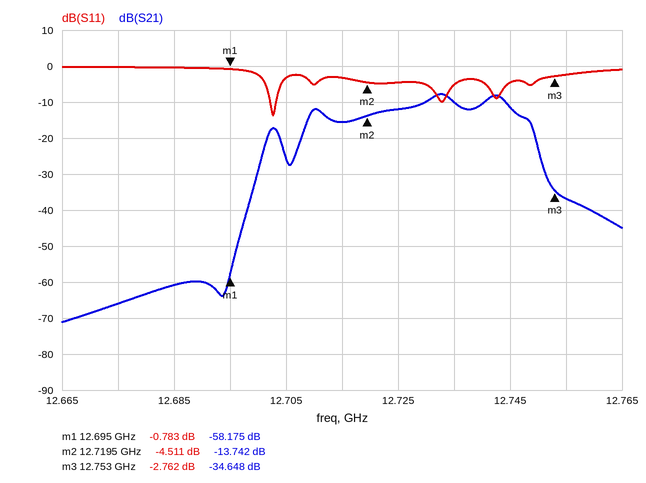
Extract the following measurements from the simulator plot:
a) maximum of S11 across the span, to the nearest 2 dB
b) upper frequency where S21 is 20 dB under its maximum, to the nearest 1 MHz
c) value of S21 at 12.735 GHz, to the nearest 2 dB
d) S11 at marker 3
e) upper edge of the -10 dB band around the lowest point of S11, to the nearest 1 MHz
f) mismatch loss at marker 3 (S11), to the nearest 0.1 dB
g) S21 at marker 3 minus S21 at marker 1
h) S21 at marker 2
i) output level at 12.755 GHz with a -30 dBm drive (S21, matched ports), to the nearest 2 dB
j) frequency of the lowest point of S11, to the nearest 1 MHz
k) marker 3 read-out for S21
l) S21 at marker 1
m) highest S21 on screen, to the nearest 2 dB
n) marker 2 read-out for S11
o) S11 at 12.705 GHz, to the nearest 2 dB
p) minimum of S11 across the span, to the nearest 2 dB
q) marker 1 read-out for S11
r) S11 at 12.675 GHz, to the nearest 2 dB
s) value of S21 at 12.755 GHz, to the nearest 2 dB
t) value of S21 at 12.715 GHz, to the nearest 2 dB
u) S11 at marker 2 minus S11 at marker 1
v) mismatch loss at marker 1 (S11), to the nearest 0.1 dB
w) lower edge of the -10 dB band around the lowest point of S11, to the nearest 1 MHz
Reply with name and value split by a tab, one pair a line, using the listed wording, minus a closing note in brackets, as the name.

maximum of S11 across the span, to the nearest 2 dB	0 dB
upper frequency where S21 is 20 dB under its maximum, to the nearest 1 MHz	12.751 GHz
value of S21 at 12.735 GHz, to the nearest 2 dB	-10 dB
S11 at marker 3	-2.762 dB
upper edge of the -10 dB band around the lowest point of S11, to the nearest 1 MHz	12.703 GHz
mismatch loss at marker 3 (S11), to the nearest 0.1 dB	3.3 dB
S21 at marker 3 minus S21 at marker 1	23.527 dB
S21 at marker 2	-13.742 dB
output level at 12.755 GHz with a -30 dBm drive (S21, matched ports), to the nearest 2 dB	-66 dBm
frequency of the lowest point of S11, to the nearest 1 MHz	12.703 GHz
marker 3 read-out for S21	-34.648 dB
S21 at marker 1	-58.175 dB
highest S21 on screen, to the nearest 2 dB	-8 dB
marker 2 read-out for S11	-4.511 dB
S11 at 12.705 GHz, to the nearest 2 dB	-4 dB
minimum of S11 across the span, to the nearest 2 dB	-14 dB
marker 1 read-out for S11	-0.783 dB
S11 at 12.675 GHz, to the nearest 2 dB	0 dB
value of S21 at 12.755 GHz, to the nearest 2 dB	-36 dB
value of S21 at 12.715 GHz, to the nearest 2 dB	-16 dB
S11 at marker 2 minus S11 at marker 1	-3.728 dB
mismatch loss at marker 1 (S11), to the nearest 0.1 dB	7.8 dB
lower edge of the -10 dB band around the lowest point of S11, to the nearest 1 MHz	12.702 GHz
